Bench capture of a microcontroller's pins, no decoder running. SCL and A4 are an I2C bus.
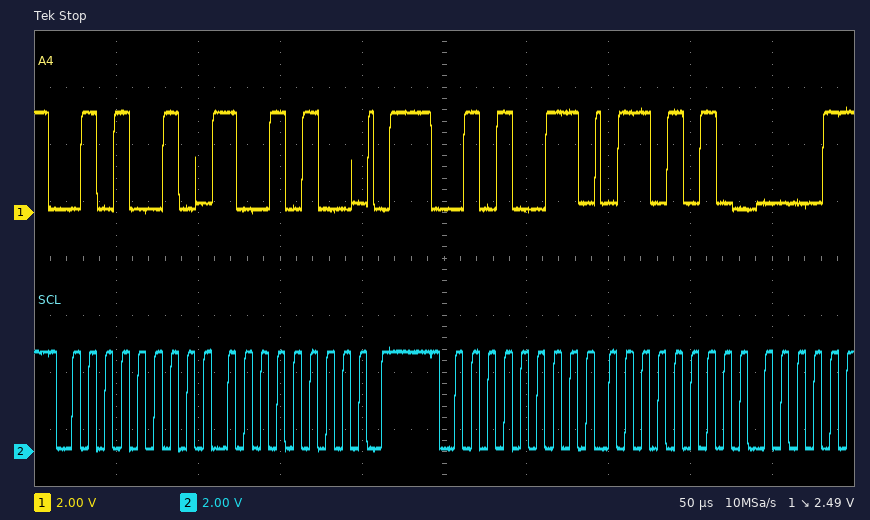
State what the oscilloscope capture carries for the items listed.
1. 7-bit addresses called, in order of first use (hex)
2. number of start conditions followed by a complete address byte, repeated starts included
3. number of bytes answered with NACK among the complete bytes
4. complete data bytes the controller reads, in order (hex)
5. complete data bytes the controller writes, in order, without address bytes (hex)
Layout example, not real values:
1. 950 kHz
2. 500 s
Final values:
1. 0x29
2. 2
3. 0
4. 6A
5. 94
